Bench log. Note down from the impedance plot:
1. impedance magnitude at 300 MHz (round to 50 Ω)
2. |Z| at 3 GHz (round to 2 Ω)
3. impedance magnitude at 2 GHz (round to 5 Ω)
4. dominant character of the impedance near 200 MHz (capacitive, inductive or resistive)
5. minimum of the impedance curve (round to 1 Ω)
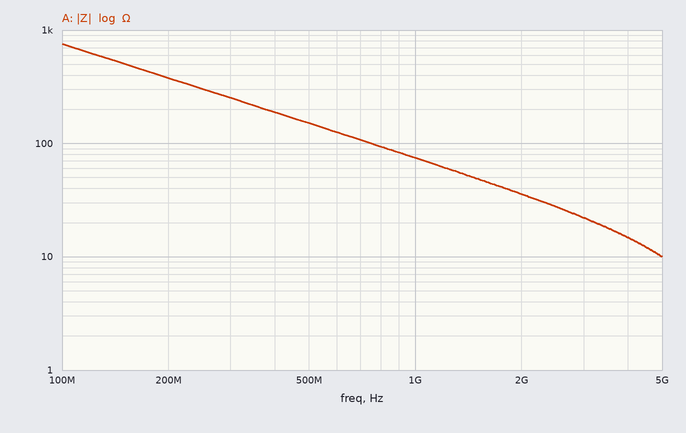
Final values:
250 Ω
22 Ω
35 Ω
capacitive
10 Ω
